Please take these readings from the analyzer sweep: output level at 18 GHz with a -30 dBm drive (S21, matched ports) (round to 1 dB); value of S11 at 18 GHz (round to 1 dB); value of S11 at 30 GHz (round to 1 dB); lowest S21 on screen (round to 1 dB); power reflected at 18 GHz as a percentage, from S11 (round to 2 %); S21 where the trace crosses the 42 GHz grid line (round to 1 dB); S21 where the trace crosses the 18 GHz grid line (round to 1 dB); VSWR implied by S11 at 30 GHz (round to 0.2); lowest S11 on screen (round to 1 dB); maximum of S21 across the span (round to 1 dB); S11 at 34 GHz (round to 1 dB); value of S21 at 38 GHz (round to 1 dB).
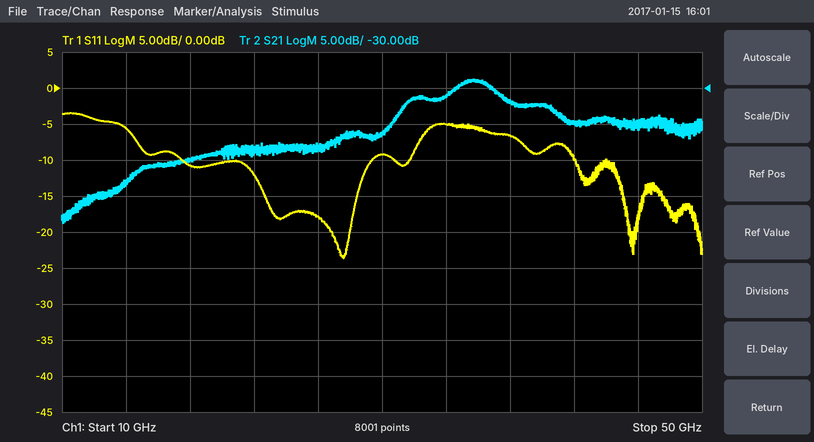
-70 dBm
-11 dB
-9 dB
-49 dB
8 %
-35 dB
-40 dB
2.0
-24 dB
-29 dB
-5 dB
-32 dB
